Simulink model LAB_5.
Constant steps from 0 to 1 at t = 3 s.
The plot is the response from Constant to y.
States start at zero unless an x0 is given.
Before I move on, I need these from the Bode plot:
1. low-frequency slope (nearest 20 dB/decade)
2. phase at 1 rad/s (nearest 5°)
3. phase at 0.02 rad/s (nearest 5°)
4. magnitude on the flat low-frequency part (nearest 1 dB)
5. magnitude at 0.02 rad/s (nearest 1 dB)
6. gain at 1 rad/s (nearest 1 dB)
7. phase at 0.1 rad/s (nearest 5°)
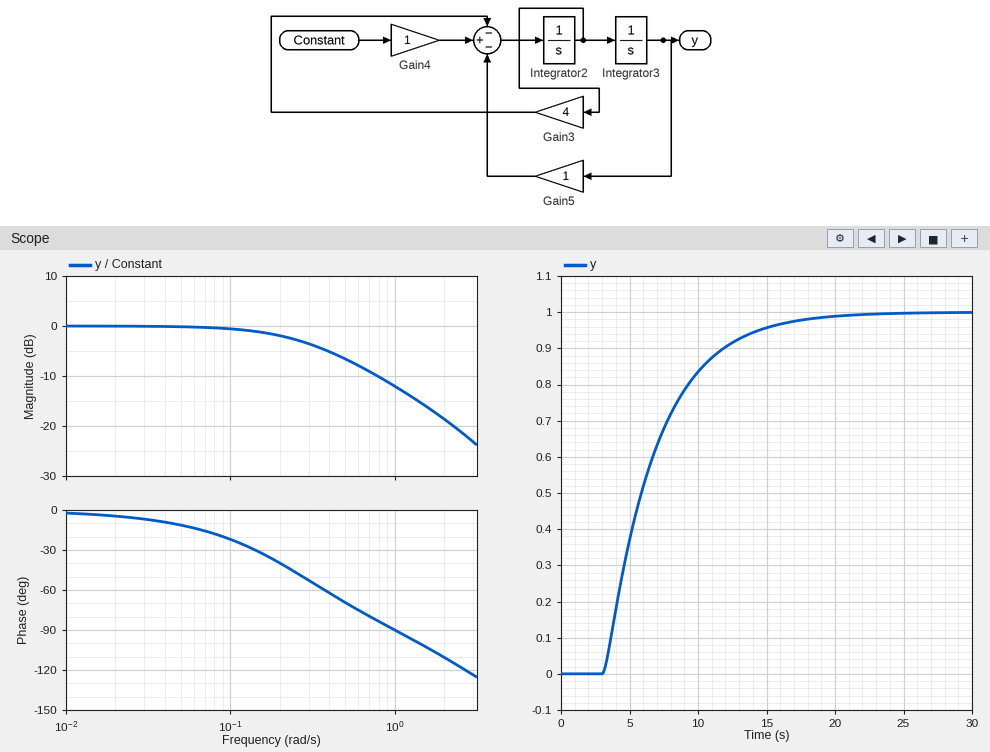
0 dB/decade
-90°
-5°
0 dB
0 dB
-12 dB
-20°
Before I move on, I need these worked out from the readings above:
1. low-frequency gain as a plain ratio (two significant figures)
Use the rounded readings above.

1.0
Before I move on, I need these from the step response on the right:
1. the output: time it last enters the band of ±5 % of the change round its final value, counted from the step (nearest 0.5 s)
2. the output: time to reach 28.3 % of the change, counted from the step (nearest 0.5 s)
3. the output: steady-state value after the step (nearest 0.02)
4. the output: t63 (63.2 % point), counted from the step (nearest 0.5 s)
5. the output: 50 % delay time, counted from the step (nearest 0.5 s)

11.5 s
1.5 s
1.00
4.0 s
3.0 s
